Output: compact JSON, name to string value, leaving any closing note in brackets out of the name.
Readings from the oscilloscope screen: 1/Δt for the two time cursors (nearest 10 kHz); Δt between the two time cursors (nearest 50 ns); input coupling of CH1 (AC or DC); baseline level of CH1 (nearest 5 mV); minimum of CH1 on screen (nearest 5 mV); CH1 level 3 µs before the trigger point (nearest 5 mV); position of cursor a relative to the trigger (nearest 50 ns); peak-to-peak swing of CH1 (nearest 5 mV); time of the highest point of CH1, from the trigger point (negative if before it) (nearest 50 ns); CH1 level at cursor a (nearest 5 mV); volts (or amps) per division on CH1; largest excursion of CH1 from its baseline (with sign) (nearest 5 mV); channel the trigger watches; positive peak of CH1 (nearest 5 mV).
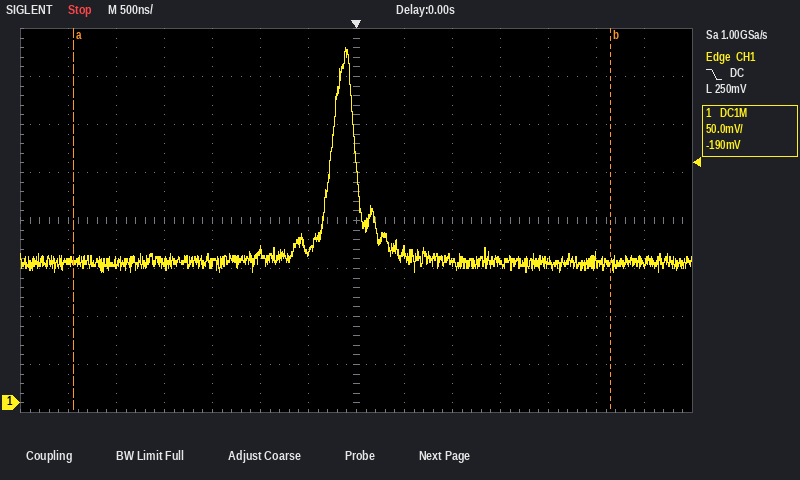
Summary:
{"1/Δt for the two time cursors": "180 kHz", "Δt between the two time cursors": "5.60 µs", "input coupling of CH1": "DC", "baseline level of CH1": "145 mV", "minimum of CH1 on screen": "135 mV", "CH1 level 3 µs before the trigger point": "145 mV", "position of cursor a relative to the trigger": "-2.95 µs", "peak-to-peak swing of CH1": "235 mV", "time of the highest point of CH1, from the trigger point (negative if before it)": "-100 ns", "CH1 level at cursor a": "145 mV", "volts (or amps) per division on CH1": "50 mV", "largest excursion of CH1 from its baseline (with sign)": "+225 mV", "channel the trigger watches": "CH1", "positive peak of CH1": "370 mV"}
